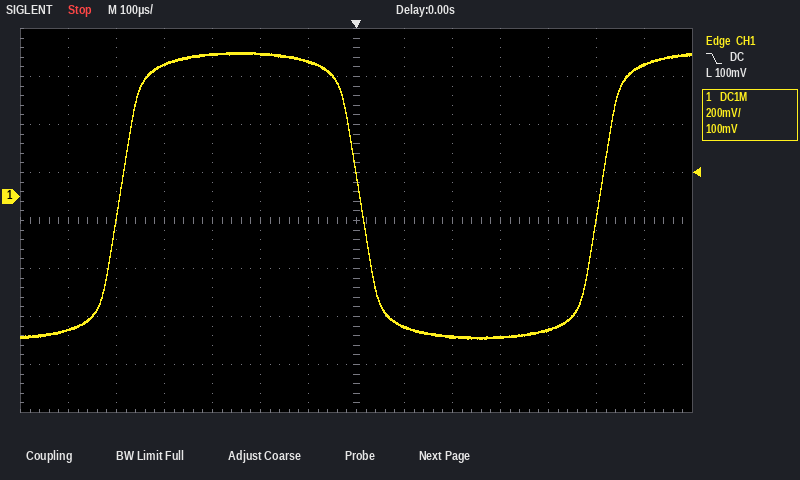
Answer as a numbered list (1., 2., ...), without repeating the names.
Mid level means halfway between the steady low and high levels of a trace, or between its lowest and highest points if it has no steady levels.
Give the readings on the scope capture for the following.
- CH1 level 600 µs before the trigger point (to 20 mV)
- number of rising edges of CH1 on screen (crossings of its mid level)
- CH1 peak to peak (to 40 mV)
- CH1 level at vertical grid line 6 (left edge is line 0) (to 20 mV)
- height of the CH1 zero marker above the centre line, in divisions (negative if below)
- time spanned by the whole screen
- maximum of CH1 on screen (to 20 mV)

1. -560 mV
2. 2
3. 1.20 V
4. 560 mV
5. +0.5 div
6. 1.4 ms
7. 600 mV
